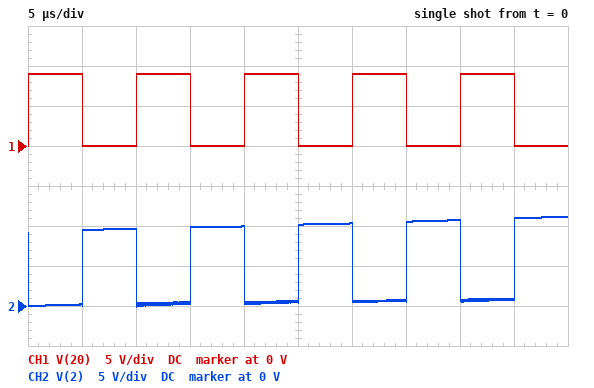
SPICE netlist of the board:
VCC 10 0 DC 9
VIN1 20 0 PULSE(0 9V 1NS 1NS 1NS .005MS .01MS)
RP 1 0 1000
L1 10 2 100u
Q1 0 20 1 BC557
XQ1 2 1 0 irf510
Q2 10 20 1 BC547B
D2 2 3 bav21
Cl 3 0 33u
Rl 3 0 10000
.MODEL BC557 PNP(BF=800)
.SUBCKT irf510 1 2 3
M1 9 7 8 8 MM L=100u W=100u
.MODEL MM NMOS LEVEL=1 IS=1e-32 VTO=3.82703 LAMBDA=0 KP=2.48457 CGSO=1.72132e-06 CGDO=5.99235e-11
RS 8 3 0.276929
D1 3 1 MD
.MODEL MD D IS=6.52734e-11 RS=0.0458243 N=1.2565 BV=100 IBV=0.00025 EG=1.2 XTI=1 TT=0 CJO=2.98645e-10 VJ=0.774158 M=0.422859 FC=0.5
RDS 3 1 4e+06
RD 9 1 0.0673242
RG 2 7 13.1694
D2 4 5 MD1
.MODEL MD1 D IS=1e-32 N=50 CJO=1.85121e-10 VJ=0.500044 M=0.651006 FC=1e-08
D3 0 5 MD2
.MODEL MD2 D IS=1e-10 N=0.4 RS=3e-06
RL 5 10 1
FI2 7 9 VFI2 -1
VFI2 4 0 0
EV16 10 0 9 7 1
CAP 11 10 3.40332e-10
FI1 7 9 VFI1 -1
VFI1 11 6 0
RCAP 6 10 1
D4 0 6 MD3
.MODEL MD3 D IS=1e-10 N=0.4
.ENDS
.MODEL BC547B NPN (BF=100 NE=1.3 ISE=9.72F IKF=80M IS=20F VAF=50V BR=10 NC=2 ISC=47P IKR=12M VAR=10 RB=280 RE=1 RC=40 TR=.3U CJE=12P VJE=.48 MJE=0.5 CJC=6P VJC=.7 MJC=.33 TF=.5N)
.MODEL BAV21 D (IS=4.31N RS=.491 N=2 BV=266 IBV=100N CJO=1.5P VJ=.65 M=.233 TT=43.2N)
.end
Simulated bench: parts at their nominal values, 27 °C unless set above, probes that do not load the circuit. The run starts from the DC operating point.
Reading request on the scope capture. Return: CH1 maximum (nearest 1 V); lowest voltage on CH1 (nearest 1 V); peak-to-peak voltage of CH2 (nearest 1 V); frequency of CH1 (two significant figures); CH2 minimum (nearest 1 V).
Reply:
9 V
0 V
11 V
100 kHz
0 V
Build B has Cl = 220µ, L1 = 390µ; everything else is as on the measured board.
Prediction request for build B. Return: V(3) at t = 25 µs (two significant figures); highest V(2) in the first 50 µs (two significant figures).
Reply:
8.4 V
9.6 V
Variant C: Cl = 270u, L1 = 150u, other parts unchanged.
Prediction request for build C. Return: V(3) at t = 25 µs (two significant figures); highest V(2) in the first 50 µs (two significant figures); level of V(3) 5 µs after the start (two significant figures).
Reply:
8.4 V
10 V
8.4 V
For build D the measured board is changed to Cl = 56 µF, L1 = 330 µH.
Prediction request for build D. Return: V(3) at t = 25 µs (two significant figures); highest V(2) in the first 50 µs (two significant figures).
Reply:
8.4 V
9.8 V
